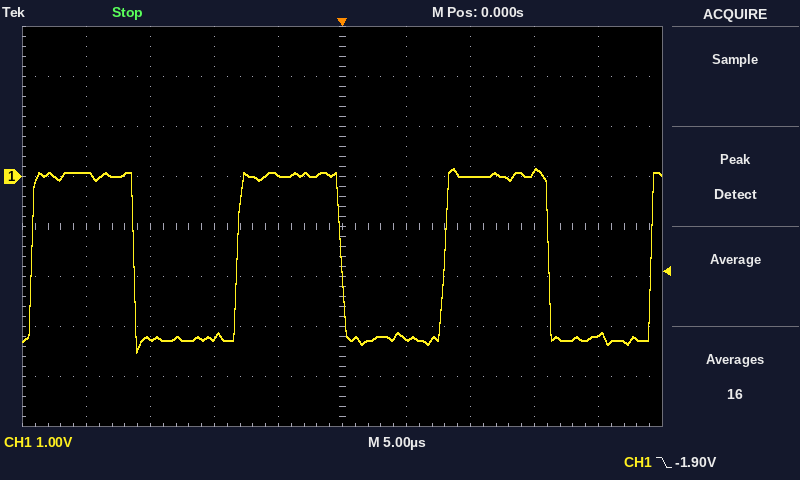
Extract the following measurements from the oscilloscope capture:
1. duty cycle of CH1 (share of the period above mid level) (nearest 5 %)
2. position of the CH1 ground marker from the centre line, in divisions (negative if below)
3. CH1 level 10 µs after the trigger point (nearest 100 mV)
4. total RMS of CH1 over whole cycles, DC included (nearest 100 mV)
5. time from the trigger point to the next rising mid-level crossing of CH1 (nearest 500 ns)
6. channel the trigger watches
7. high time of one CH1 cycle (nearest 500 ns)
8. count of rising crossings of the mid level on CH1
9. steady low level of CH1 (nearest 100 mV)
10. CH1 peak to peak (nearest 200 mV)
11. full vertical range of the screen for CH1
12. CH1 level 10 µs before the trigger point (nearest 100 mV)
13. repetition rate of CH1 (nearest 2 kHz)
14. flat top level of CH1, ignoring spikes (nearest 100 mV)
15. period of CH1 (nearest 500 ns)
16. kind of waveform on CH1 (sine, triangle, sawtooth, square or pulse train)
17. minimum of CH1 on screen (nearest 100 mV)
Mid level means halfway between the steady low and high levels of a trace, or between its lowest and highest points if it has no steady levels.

50 %
+1.0 div
0.0 V
2.3 V
8.0 µs
CH1
8.0 µs
4
-3.3 V
3.6 V
8 V
-3.2 V
62 kHz
0.0 V
16.0 µs
square
-3.5 V
